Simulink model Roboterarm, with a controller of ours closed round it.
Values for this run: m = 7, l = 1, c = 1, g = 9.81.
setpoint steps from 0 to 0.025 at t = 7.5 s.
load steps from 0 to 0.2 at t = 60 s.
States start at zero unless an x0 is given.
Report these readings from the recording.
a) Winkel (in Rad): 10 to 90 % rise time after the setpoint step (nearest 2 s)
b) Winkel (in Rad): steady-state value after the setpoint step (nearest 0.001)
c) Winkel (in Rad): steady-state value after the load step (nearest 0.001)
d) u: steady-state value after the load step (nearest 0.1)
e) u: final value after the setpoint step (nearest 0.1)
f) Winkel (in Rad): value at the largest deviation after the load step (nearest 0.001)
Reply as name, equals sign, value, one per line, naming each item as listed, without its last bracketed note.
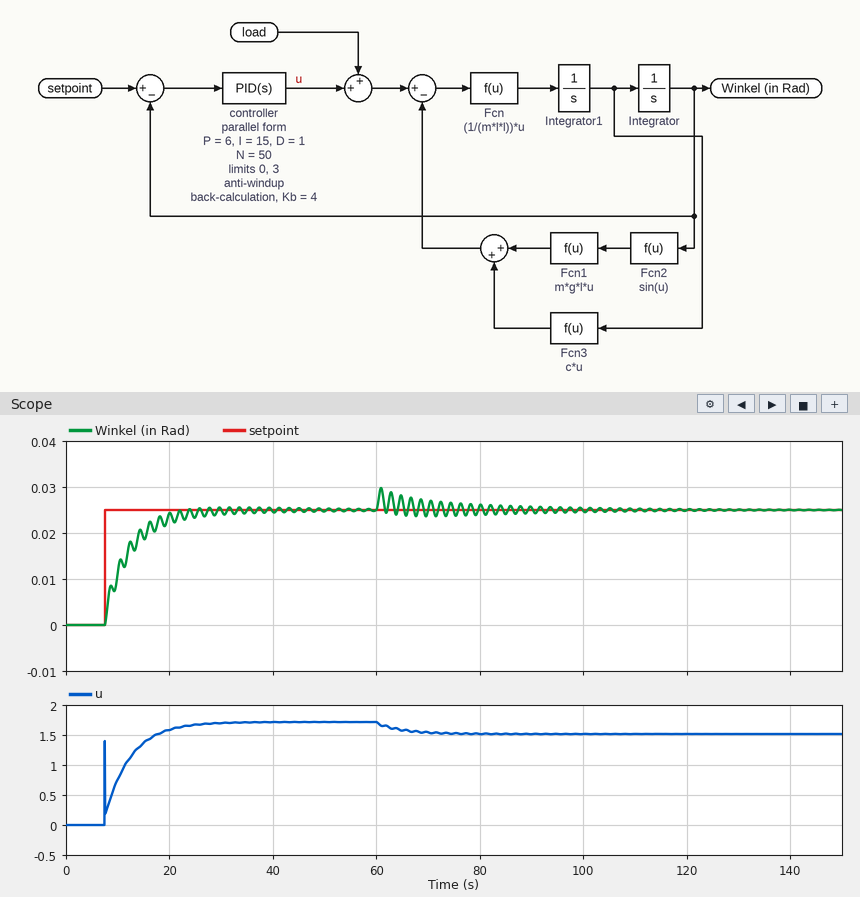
Winkel (in Rad): 10 to 90 % rise time after the setpoint step = 10 s
Winkel (in Rad): steady-state value after the setpoint step = 0.025
Winkel (in Rad): steady-state value after the load step = 0.025
u: steady-state value after the load step = 1.5
u: final value after the setpoint step = 1.7
Winkel (in Rad): value at the largest deviation after the load step = 0.030
